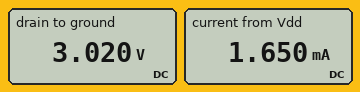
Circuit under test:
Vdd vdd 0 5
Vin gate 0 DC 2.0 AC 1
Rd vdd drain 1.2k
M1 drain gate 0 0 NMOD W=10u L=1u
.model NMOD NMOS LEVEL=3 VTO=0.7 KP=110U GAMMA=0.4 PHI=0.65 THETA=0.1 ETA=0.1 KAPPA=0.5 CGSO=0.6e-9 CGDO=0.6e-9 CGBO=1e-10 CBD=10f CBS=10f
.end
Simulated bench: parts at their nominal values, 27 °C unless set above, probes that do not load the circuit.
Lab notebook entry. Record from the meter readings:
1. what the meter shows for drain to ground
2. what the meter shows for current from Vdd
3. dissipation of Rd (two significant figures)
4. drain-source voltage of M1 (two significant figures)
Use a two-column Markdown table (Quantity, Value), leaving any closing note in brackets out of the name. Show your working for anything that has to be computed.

| Quantity | Value |
|---|---|
| what the meter shows for drain to ground | 3.020 V |
| what the meter shows for current from Vdd | 1.650 mA |
| dissipation of Rd | (5 V - 3.02 V)^2 / 1.2 kΩ = 3.3 mW |
| drain-source voltage of M1 | 3.02 V = 3.0 V |
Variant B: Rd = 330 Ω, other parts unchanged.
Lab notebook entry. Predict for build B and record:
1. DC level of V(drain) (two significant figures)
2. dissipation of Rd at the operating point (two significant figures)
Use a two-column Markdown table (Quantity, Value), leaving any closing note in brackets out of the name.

| Quantity | Value |
|---|---|
| DC level of V(drain) | 4.3 V |
| dissipation of Rd at the operating point | 1.5 mW |
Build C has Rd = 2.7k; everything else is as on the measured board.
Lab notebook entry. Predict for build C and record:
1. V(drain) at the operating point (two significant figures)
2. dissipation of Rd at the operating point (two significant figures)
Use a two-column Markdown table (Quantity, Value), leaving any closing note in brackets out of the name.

| Quantity | Value |
|---|---|
| V(drain) at the operating point | 1.7 V |
| dissipation of Rd at the operating point | 4.0 mW |
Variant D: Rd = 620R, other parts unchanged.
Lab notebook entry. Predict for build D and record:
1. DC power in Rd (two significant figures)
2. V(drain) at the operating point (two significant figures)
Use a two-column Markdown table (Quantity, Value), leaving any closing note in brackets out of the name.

| Quantity | Value |
|---|---|
| DC power in Rd | 2.3 mW |
| V(drain) at the operating point | 3.8 V |
